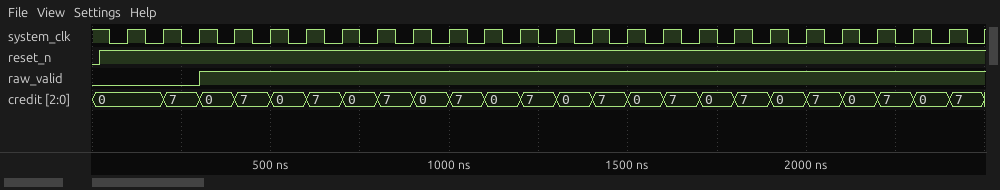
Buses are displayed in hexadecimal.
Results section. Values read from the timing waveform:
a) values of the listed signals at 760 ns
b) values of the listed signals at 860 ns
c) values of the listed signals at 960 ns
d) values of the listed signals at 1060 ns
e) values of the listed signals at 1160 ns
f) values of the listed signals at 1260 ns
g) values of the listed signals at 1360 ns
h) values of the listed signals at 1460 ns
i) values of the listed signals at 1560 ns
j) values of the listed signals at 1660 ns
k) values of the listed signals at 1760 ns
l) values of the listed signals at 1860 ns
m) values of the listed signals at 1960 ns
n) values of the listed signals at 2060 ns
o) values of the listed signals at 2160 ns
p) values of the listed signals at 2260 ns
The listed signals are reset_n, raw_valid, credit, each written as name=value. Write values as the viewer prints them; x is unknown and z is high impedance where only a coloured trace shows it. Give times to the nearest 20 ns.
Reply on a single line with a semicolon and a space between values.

reset_n=1, raw_valid=1, credit=0; reset_n=1, raw_valid=1, credit=7; reset_n=1, raw_valid=1, credit=0; reset_n=1, raw_valid=1, credit=7; reset_n=1, raw_valid=1, credit=0; reset_n=1, raw_valid=1, credit=7; reset_n=1, raw_valid=1, credit=0; reset_n=1, raw_valid=1, credit=7; reset_n=1, raw_valid=1, credit=0; reset_n=1, raw_valid=1, credit=7; reset_n=1, raw_valid=1, credit=0; reset_n=1, raw_valid=1, credit=7; reset_n=1, raw_valid=1, credit=0; reset_n=1, raw_valid=1, credit=7; reset_n=1, raw_valid=1, credit=0; reset_n=1, raw_valid=1, credit=7
